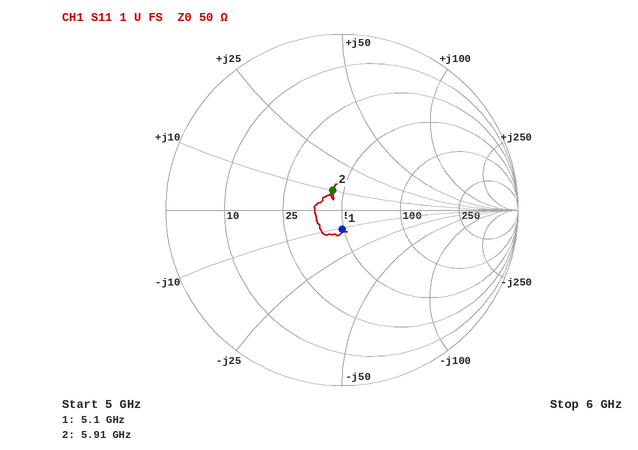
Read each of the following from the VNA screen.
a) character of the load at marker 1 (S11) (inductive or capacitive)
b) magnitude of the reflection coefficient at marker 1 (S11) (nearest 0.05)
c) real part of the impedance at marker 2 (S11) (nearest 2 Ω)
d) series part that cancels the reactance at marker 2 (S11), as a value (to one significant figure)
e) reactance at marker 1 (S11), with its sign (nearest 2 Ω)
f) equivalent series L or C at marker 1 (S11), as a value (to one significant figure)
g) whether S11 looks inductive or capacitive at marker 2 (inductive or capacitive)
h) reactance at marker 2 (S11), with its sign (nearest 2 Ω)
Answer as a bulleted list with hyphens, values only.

- capacitive
- 0.10
- 44 Ω
- 3 pF
- -10 Ω
- 3 pF
- inductive
- +10 Ω
